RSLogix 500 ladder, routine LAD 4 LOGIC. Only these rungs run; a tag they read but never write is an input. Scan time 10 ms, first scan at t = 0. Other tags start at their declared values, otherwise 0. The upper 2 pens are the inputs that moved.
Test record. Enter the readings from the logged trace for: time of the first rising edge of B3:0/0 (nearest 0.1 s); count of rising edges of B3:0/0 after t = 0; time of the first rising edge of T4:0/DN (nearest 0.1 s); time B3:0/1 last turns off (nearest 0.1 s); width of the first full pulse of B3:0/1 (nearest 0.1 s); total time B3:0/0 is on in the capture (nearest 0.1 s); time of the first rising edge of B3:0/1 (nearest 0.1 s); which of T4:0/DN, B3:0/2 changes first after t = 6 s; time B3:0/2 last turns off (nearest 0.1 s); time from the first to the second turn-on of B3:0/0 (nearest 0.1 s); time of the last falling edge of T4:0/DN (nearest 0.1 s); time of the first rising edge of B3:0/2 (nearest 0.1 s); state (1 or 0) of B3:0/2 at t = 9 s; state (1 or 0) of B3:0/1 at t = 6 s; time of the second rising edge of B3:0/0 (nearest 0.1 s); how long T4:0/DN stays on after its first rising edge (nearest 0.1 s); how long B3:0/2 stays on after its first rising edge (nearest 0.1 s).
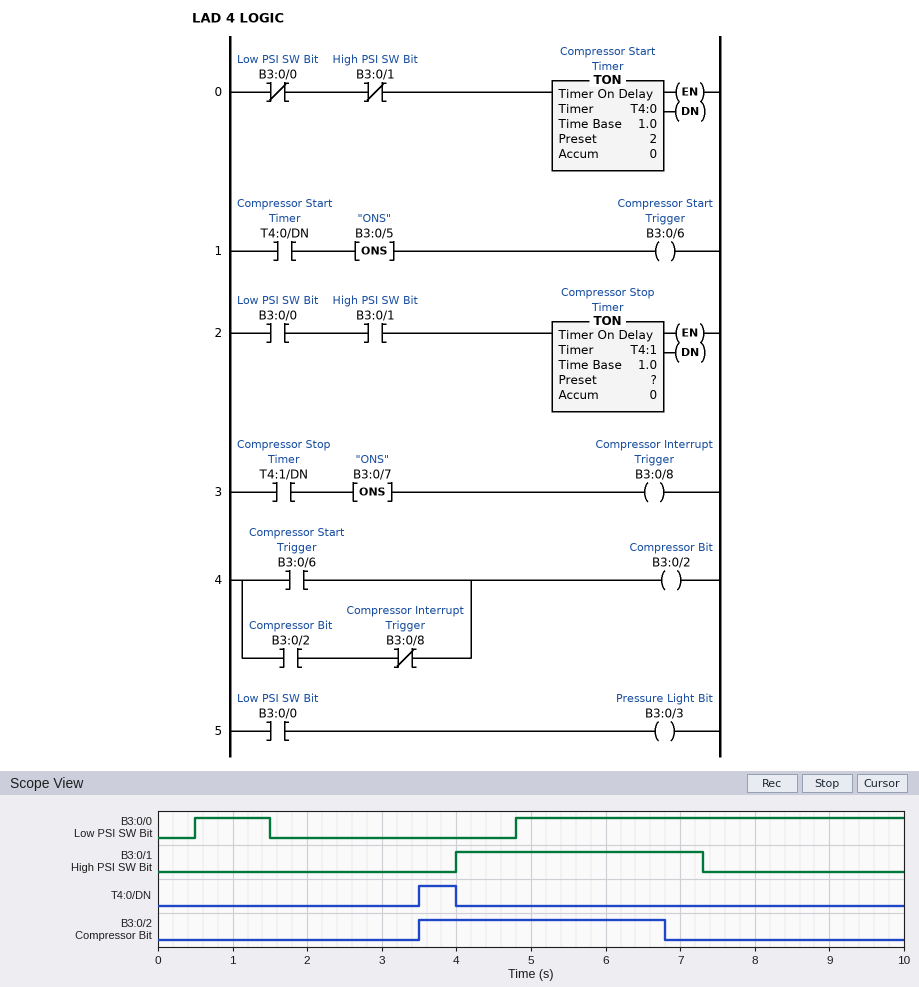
0.5 s
2
3.5 s
7.3 s
3.3 s
6.2 s
4.0 s
B3:0/2
6.8 s
4.3 s
4.0 s
3.5 s
0
1
4.8 s
0.5 s
3.3 s
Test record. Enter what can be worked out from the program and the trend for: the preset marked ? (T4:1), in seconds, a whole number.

2 s
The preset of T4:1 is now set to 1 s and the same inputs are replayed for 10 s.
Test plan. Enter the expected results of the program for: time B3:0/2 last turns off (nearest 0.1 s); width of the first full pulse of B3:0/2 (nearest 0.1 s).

5.8 s
2.3 s
